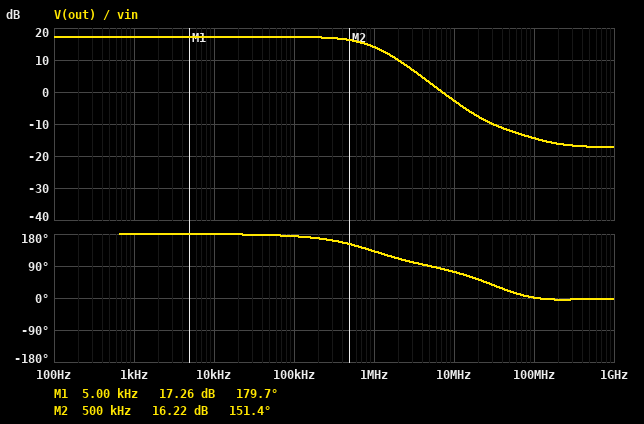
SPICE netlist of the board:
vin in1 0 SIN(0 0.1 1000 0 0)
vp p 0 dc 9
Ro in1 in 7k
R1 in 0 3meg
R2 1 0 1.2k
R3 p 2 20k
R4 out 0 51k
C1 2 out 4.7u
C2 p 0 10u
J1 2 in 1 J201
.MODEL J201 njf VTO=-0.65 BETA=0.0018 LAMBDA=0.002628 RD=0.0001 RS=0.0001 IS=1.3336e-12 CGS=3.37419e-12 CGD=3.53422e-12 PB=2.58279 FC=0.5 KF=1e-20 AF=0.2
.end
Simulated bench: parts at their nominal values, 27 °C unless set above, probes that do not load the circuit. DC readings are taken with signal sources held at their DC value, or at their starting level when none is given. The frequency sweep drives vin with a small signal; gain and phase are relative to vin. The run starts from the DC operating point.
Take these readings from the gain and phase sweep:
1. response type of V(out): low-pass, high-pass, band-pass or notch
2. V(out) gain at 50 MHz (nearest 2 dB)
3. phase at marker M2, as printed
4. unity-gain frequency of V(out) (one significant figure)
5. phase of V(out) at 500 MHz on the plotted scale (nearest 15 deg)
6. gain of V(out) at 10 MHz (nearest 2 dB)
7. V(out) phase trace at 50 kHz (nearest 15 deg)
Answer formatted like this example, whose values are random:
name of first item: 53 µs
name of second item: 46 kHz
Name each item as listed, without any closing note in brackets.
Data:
response type of V(out): low-pass, high-pass, band-pass or notch: low-pass
V(out) gain at 50 MHz: -12 dB
phase at marker M2, as printed: 151.4 deg
unity-gain frequency of V(out): 7 MHz
phase of V(out) at 500 MHz on the plotted scale: 0 deg
gain of V(out) at 10 MHz: -2 dB
V(out) phase trace at 50 kHz: 180 deg
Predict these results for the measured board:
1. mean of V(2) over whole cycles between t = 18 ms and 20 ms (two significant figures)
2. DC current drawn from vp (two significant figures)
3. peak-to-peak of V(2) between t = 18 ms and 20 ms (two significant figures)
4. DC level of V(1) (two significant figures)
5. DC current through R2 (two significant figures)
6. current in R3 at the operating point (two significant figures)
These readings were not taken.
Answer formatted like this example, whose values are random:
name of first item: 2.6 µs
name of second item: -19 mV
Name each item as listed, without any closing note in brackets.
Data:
mean of V(2) over whole cycles between t = 18 ms and 20 ms: 4.2 V
DC current drawn from vp: 240 µA
peak-to-peak of V(2) between t = 18 ms and 20 ms: 1.5 V
DC level of V(1): 290 mV
DC current through R2: 240 µA
current in R3 at the operating point: 240 µA
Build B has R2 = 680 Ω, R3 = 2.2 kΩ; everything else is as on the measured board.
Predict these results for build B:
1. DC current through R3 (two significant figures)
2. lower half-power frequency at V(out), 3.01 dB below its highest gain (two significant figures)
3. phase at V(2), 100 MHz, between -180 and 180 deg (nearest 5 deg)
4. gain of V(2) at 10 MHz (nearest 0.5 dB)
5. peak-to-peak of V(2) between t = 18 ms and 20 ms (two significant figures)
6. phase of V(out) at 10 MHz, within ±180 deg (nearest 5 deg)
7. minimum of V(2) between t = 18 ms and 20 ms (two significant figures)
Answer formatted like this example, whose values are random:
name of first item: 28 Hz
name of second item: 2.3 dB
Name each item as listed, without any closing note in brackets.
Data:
DC current through R3: 330 µA
lower half-power frequency at V(out), 3.01 dB below its highest gain: 640 mHz
phase at V(2), 100 MHz, between -180 and 180 deg: 20 deg
gain of V(2) at 10 MHz: -5.5 dB
peak-to-peak of V(2) between t = 18 ms and 20 ms: 320 mV
phase of V(out) at 10 MHz, within ±180 deg: 95 deg
minimum of V(2) between t = 18 ms and 20 ms: 8.1 V
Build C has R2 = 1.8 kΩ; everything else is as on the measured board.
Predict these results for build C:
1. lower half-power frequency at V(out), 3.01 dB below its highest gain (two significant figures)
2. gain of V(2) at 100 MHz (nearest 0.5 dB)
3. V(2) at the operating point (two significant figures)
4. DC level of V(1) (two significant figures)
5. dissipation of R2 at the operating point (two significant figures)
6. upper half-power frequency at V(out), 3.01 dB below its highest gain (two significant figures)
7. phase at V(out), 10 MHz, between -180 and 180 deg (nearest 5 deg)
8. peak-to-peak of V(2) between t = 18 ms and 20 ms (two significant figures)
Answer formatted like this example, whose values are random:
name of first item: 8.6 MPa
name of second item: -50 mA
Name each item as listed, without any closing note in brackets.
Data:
lower half-power frequency at V(out), 3.01 dB below its highest gain: 480 mHz
gain of V(2) at 100 MHz: -12.5 dB
V(2) at the operating point: 5.3 V
DC level of V(1): 330 mV
dissipation of R2 at the operating point: 61 µW
upper half-power frequency at V(out), 3.01 dB below its highest gain: 1.3 MHz
phase at V(out), 10 MHz, between -180 and 180 deg: 70 deg
peak-to-peak of V(2) between t = 18 ms and 20 ms: 1.1 V
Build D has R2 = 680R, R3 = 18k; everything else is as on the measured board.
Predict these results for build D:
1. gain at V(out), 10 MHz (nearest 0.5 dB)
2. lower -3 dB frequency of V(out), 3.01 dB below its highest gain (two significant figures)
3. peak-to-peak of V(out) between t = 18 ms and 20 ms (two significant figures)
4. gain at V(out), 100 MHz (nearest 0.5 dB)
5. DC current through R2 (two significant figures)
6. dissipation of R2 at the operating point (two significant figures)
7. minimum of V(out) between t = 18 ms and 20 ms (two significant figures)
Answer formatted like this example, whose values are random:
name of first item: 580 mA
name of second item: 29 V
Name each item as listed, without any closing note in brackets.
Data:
gain at V(out), 10 MHz: -3.0 dB
lower -3 dB frequency of V(out), 3.01 dB below its highest gain: 490 mHz
peak-to-peak of V(out) between t = 18 ms and 20 ms: 2.0 V
gain at V(out), 100 MHz: -17.0 dB
DC current through R2: 330 µA
dissipation of R2 at the operating point: 74 µW
minimum of V(out) between t = 18 ms and 20 ms: -1.0 V
